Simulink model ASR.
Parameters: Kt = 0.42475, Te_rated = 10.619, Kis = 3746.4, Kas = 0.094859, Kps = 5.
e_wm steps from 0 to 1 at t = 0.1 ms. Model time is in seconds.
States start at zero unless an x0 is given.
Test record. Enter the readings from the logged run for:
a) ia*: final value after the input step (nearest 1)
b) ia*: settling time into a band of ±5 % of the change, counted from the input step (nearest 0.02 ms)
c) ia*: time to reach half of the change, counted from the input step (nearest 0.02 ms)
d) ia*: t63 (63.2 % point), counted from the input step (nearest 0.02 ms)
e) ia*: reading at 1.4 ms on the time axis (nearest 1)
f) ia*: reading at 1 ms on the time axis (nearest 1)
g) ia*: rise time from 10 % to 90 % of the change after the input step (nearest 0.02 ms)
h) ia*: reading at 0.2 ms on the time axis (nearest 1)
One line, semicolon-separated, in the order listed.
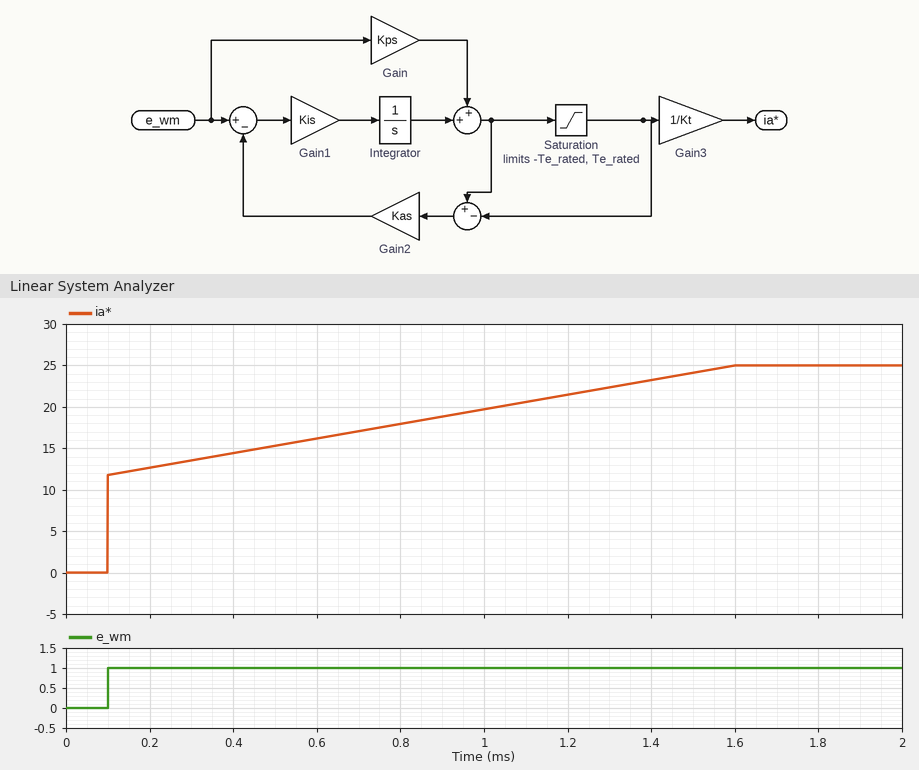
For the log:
25; 1.36 ms; 0.08 ms; 0.46 ms; 23; 20; 1.22 ms; 13
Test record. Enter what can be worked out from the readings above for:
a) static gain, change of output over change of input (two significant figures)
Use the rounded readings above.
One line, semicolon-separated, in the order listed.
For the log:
25
